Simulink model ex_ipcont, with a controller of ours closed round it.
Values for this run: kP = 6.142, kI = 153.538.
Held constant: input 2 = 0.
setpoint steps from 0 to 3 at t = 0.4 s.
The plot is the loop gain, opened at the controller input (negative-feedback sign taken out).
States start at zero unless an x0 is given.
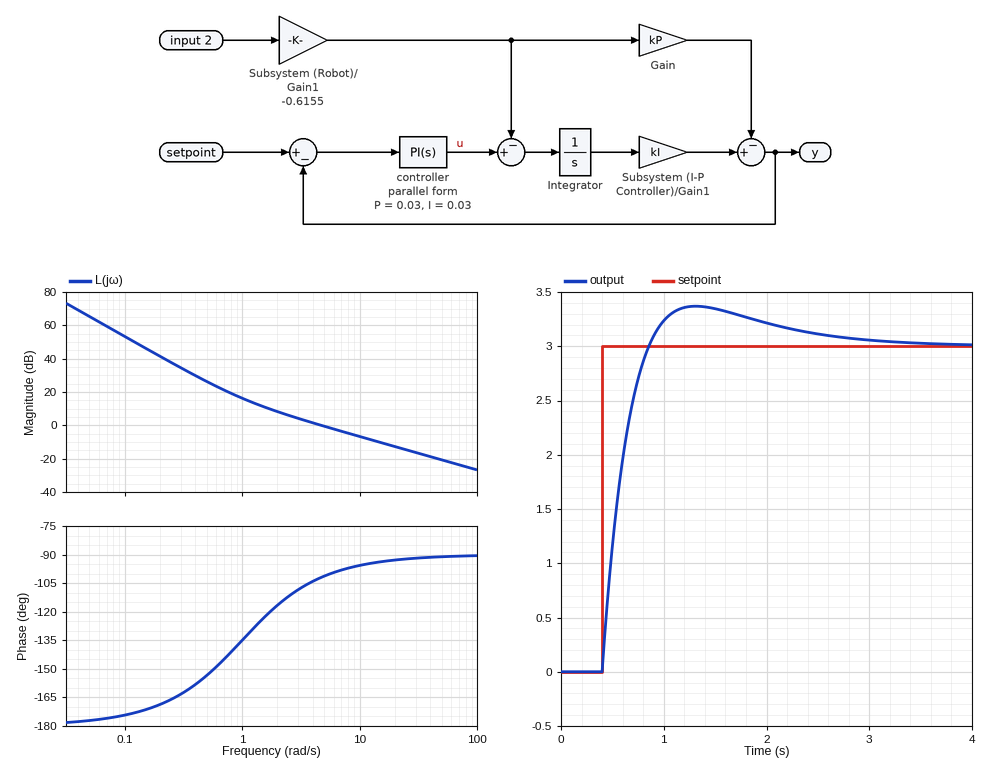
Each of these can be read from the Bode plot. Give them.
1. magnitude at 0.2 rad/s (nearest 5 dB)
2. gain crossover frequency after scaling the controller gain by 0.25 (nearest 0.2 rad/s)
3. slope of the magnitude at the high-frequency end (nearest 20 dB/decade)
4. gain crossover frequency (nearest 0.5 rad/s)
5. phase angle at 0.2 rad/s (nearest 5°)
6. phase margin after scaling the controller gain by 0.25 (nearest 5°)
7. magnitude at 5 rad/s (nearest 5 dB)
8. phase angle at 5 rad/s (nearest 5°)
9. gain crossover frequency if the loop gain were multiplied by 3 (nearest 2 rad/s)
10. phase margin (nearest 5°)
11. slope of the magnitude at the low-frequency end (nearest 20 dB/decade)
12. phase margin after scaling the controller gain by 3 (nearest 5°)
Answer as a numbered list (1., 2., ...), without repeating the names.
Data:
1. 40 dB
2. 1.4 rad/s
3. -20 dB/decade
4. 4.5 rad/s
5. -170°
6. 55°
7. 0 dB
8. -100°
9. 14 rad/s
10. 80°
11. -40 dB/decade
12. 85°
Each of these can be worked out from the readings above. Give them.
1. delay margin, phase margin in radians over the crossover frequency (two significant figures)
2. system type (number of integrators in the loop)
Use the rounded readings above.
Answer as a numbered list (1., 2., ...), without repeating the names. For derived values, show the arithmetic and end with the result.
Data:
1. 80 × π / 180 / 4.5 = 0.31 s
2. 2
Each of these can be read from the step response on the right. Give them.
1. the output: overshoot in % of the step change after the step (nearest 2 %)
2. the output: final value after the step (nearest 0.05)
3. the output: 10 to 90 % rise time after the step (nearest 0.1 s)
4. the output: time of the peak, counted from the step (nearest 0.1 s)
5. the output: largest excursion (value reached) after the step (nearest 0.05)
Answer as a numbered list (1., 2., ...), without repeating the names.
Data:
1. 12 %
2. 3.00
3. 0.3 s
4. 0.9 s
5. 3.35
